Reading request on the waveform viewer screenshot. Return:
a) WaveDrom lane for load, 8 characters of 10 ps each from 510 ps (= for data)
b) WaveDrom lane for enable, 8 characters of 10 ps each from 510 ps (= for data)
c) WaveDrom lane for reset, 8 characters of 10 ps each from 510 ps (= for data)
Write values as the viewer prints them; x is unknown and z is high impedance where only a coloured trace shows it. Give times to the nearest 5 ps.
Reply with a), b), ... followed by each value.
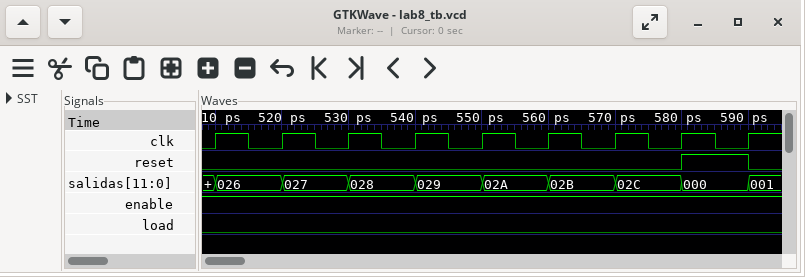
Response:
a) {name: 'load', wave: '0.......'}
b) {name: 'enable', wave: '1.......'}
c) {name: 'reset', wave: '0......1'}
